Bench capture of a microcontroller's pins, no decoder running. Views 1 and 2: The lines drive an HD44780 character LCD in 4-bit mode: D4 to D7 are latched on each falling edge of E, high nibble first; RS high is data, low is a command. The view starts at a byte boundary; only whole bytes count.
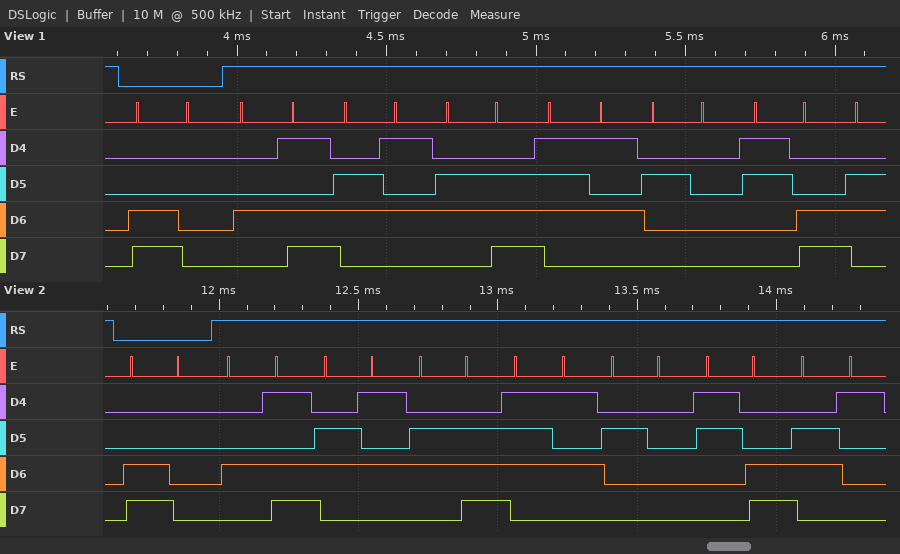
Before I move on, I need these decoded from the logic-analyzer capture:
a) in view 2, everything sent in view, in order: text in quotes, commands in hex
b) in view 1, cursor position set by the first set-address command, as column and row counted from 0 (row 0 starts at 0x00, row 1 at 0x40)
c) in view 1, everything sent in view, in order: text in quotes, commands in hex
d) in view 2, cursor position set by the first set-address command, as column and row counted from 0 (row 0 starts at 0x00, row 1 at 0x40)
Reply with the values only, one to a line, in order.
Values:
0xC0 "Menu <a"
column 0, row 1
0xC0 "Menu <"
column 0, row 1
